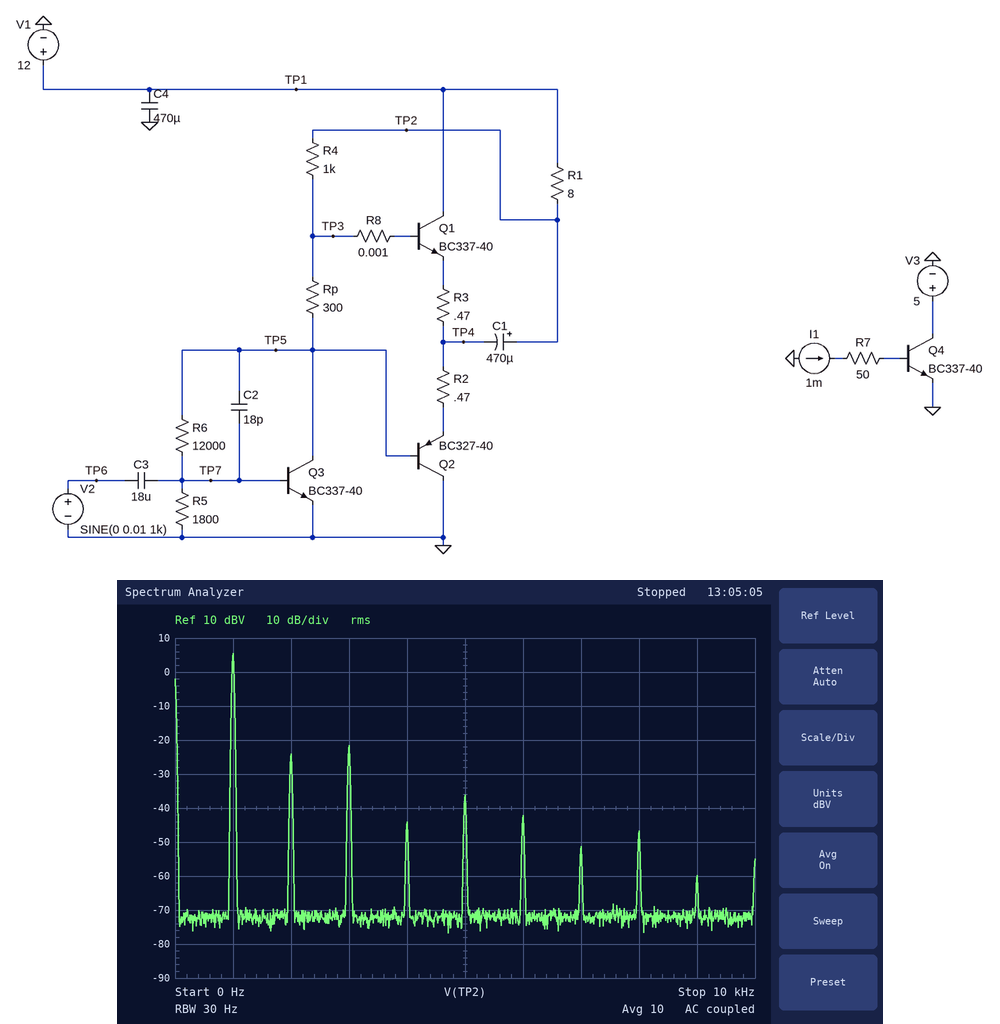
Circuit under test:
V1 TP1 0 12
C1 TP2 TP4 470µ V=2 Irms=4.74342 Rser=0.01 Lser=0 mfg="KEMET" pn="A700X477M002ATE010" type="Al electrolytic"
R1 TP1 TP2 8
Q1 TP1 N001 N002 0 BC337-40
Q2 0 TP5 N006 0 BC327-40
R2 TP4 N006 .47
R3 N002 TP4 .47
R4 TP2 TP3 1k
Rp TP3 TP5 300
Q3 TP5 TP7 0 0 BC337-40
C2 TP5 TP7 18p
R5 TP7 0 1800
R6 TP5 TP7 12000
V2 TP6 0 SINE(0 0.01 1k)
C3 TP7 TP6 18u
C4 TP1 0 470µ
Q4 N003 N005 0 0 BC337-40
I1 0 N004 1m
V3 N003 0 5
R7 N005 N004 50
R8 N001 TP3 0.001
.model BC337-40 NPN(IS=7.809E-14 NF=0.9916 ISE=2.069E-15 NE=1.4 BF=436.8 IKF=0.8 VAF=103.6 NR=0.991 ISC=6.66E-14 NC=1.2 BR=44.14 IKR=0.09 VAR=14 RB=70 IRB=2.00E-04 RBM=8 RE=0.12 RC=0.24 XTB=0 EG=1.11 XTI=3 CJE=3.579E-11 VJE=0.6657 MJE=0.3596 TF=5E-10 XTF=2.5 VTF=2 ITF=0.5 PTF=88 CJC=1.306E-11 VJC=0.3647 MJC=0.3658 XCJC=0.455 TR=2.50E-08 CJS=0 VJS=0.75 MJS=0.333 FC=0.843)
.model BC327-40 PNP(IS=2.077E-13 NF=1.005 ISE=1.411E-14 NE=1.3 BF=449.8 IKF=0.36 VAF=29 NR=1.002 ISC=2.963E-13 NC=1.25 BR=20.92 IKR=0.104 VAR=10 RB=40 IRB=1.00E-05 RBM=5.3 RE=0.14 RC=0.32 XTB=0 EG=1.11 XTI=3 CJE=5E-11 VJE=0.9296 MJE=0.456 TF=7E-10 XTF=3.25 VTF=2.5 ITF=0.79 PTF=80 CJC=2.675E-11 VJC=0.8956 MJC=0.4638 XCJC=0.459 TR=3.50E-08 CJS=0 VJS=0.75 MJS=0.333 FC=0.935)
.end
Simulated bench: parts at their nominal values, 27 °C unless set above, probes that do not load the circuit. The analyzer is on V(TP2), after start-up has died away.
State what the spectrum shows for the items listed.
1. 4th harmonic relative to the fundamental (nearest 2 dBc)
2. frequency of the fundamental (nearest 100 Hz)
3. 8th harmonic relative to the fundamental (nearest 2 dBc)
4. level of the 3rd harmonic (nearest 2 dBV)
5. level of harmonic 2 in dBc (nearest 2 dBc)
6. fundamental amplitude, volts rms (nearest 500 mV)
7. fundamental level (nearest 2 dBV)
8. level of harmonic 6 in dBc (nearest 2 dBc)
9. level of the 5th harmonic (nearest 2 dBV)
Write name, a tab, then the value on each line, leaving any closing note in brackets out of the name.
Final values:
4th harmonic relative to the fundamental	-50 dBc
frequency of the fundamental	1.0 kHz
8th harmonic relative to the fundamental	-52 dBc
level of the 3rd harmonic	-22 dBV
level of harmonic 2 in dBc	-30 dBc
fundamental amplitude, volts rms	2.0 V
fundamental level	6 dBV
level of harmonic 6 in dBc	-48 dBc
level of the 5th harmonic	-36 dBV
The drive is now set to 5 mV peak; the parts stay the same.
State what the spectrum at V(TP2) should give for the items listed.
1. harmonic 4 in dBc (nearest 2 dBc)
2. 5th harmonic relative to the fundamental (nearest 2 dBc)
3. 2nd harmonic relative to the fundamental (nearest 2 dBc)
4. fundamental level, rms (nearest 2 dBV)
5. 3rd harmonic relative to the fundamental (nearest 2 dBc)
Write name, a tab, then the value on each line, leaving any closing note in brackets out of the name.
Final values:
harmonic 4 in dBc	-44 dBc
5th harmonic relative to the fundamental	-56 dBc
2nd harmonic relative to the fundamental	-50 dBc
fundamental level, rms	0 dBV
3rd harmonic relative to the fundamental	-36 dBc
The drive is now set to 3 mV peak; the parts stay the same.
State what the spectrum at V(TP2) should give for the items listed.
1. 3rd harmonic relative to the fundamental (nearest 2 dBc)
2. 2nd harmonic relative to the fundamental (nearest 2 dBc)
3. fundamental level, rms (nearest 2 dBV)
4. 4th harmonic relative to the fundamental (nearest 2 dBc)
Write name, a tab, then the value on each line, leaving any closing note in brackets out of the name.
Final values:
3rd harmonic relative to the fundamental	-48 dBc
2nd harmonic relative to the fundamental	-40 dBc
fundamental level, rms	-4 dBV
4th harmonic relative to the fundamental	-58 dBc
